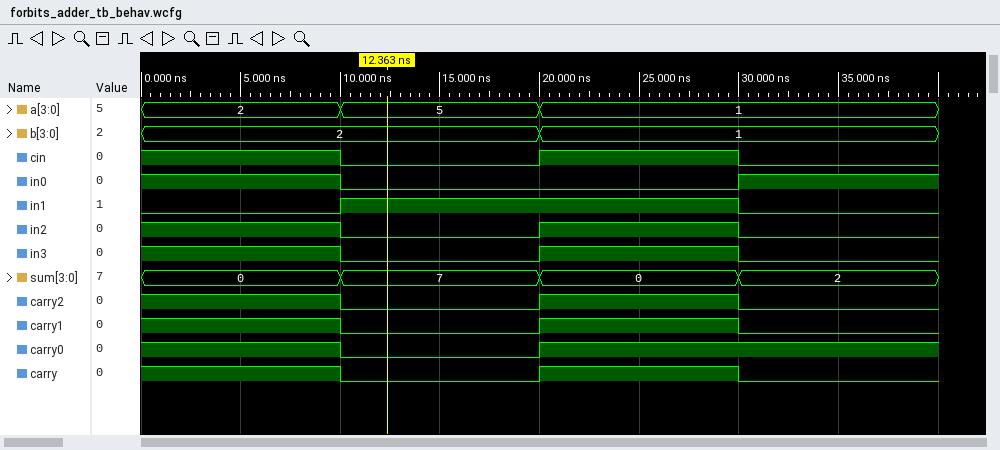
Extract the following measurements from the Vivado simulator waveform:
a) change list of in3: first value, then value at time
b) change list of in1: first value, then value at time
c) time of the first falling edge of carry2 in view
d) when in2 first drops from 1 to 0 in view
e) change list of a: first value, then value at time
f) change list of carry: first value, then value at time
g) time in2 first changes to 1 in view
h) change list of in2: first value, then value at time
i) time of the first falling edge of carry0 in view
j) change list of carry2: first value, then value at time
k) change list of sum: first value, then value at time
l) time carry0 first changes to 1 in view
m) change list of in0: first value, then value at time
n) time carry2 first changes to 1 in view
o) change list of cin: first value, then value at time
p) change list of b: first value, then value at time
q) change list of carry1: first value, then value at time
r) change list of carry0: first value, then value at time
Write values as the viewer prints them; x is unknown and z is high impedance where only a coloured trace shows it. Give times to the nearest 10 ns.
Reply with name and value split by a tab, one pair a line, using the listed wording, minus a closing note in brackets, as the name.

change list of in3: first value, then value at time	1, 0 at 10 ns, 1 at 20 ns, 0 at 30 ns
change list of in1: first value, then value at time	0, 1 at 10 ns, 0 at 30 ns
time of the first falling edge of carry2 in view	10 ns
when in2 first drops from 1 to 0 in view	10 ns
change list of a: first value, then value at time	2, 5 at 10 ns, 1 at 20 ns
change list of carry: first value, then value at time	1, 0 at 10 ns, 1 at 20 ns, 0 at 30 ns
time in2 first changes to 1 in view	20 ns
change list of in2: first value, then value at time	1, 0 at 10 ns, 1 at 20 ns, 0 at 30 ns
time of the first falling edge of carry0 in view	10 ns
change list of carry2: first value, then value at time	1, 0 at 10 ns, 1 at 20 ns, 0 at 30 ns
change list of sum: first value, then value at time	0, 7 at 10 ns, 0 at 20 ns, 2 at 30 ns
time carry0 first changes to 1 in view	20 ns
change list of in0: first value, then value at time	1, 0 at 10 ns, 1 at 30 ns
time carry2 first changes to 1 in view	20 ns
change list of cin: first value, then value at time	1, 0 at 10 ns, 1 at 20 ns, 0 at 30 ns
change list of b: first value, then value at time	2, 1 at 20 ns
change list of carry1: first value, then value at time	1, 0 at 10 ns, 1 at 20 ns, 0 at 30 ns
change list of carry0: first value, then value at time	1, 0 at 10 ns, 1 at 20 ns
